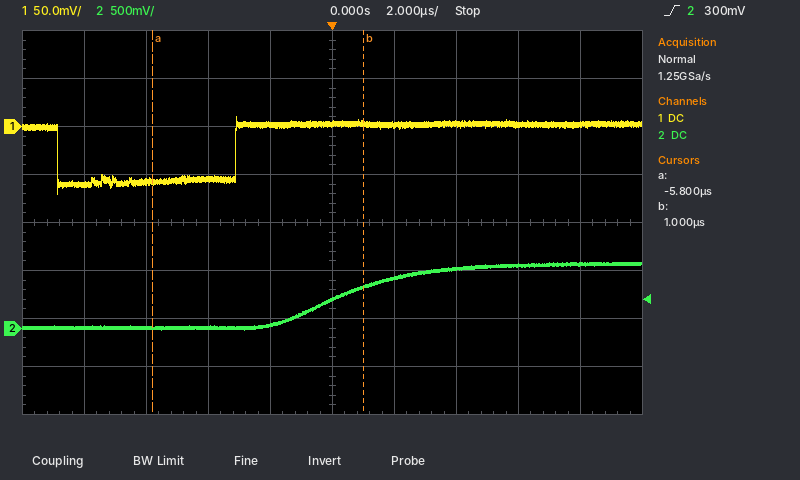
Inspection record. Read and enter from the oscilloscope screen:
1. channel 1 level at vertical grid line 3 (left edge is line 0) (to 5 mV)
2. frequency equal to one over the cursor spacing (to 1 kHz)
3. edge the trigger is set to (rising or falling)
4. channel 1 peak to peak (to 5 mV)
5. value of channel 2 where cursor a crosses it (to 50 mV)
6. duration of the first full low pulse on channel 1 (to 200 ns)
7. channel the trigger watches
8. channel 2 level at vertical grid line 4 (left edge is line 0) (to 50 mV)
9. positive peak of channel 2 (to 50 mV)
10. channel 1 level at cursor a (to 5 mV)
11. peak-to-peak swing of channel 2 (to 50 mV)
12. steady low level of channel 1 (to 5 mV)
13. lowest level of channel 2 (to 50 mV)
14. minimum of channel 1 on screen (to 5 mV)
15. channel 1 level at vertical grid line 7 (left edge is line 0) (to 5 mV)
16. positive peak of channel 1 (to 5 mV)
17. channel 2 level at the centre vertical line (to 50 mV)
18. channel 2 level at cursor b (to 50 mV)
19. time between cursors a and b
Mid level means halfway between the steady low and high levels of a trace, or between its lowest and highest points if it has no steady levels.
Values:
-55 mV
147 kHz
rising
80 mV
0 mV
5.8 µs
channel 2
50 mV
700 mV
-55 mV
700 mV
-55 mV
0 mV
-70 mV
5 mV
10 mV
300 mV
450 mV
6.8 µs
